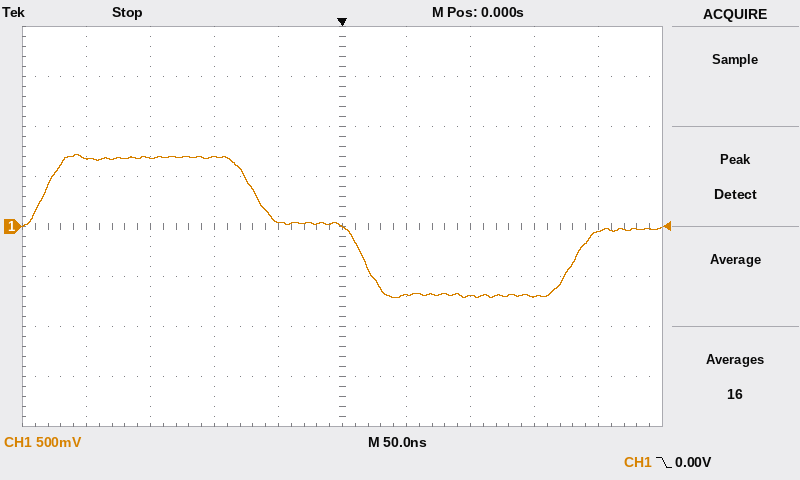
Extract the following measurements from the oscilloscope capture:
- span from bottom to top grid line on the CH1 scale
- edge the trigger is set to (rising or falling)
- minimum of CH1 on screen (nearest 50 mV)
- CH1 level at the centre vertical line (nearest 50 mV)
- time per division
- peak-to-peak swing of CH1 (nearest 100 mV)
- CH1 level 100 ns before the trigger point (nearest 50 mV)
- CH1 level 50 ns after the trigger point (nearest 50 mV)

4 V
falling
-700 mV
0 mV
50 ns
1.40 V
700 mV
-700 mV
